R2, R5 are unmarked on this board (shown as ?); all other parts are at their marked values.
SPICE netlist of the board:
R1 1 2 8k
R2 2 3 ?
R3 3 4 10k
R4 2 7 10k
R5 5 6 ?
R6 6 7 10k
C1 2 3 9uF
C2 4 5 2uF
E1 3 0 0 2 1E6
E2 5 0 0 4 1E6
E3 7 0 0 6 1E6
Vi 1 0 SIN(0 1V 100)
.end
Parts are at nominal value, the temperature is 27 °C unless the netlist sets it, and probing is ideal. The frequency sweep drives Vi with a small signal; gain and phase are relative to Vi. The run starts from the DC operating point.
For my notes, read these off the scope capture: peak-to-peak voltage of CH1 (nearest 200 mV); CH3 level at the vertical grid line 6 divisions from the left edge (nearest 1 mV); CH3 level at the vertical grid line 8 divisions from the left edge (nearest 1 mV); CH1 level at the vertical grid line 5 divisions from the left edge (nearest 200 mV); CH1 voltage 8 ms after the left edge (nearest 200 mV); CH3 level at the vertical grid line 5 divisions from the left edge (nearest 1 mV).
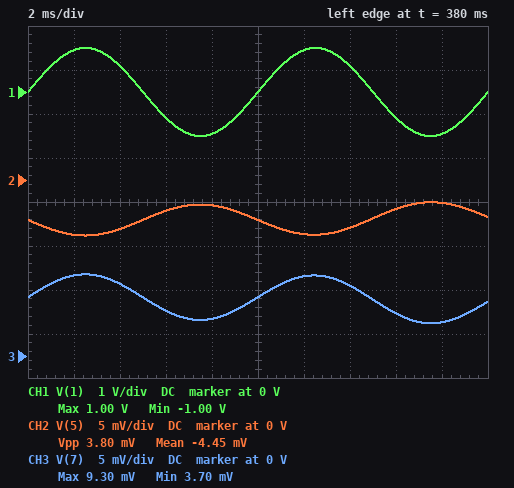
2.0 V
9 mV
5 mV
0 V
-1.0 V
7 mV
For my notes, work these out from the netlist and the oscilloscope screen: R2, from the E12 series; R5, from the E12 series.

10 kΩ
6.8 kΩ
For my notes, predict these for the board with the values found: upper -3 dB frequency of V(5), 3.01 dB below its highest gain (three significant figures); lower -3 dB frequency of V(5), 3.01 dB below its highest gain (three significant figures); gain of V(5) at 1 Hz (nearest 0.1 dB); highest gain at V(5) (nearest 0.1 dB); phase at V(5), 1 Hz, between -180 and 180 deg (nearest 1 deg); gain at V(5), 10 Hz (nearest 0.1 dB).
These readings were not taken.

5.20 Hz
3.35 Hz
-1.0 dB
7.0 dB
-5 deg
-13.3 dB
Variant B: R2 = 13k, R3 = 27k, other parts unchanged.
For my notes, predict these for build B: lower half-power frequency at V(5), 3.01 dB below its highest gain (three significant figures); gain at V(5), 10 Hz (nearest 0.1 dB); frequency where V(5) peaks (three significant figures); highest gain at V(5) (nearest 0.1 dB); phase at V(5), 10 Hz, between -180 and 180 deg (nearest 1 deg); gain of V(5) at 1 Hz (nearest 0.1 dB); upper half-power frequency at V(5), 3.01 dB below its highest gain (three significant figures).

1.76 Hz
-23.1 dB
2.60 Hz
5.0 dB
-172 deg
-0.4 dB
3.22 Hz
